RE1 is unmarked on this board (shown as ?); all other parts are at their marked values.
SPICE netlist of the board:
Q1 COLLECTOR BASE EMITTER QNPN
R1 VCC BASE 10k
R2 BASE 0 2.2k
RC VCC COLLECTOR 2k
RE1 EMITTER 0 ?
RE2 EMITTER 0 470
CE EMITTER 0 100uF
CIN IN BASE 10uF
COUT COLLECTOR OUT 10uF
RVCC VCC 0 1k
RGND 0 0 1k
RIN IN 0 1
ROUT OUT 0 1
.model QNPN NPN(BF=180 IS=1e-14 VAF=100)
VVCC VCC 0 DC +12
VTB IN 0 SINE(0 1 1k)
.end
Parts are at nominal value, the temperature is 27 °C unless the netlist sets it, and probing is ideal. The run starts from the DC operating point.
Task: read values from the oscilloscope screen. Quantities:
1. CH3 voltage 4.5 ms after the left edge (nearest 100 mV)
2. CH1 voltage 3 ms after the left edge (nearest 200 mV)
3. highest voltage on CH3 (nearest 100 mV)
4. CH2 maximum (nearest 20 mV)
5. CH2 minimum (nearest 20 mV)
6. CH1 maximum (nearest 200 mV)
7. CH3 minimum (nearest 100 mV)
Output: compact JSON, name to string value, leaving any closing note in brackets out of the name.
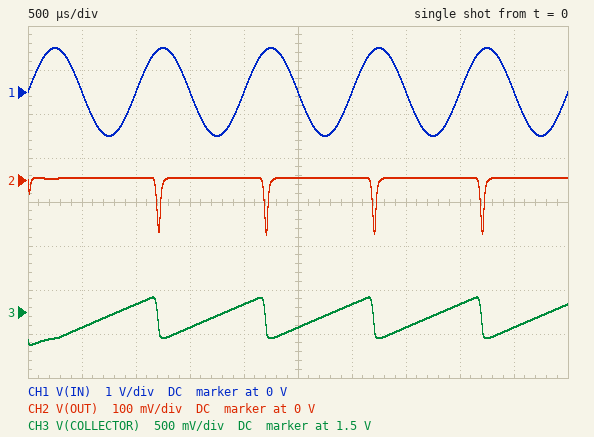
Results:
{"CH3 voltage 4.5 ms after the left edge": "1.3 V", "CH1 voltage 3 ms after the left edge": "0 V", "highest voltage on CH3": "1.7 V", "CH2 maximum": "0 V", "CH2 minimum": "-120 mV", "CH1 maximum": "1.0 V", "CH3 minimum": "1.1 V"}
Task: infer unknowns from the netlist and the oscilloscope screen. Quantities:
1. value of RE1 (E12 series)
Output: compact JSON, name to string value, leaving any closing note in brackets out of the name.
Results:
{"value of RE1": "330 Ω"}
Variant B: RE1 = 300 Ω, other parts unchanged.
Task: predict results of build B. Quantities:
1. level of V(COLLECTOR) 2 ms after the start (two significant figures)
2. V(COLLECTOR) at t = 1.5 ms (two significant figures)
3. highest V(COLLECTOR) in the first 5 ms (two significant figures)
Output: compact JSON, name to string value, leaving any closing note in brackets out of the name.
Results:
{"level of V(COLLECTOR) 2 ms after the start": "1.5 V", "V(COLLECTOR) at t = 1.5 ms": "1.3 V", "highest V(COLLECTOR) in the first 5 ms": "1.6 V"}
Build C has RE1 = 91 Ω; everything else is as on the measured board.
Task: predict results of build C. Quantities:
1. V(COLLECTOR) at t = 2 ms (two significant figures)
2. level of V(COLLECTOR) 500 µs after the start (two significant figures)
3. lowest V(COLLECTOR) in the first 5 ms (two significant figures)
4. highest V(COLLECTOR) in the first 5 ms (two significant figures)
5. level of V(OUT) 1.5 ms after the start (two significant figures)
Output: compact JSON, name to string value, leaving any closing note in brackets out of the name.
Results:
{"V(COLLECTOR) at t = 2 ms": "990 mV", "level of V(COLLECTOR) 500 µs after the start": "720 mV", "lowest V(COLLECTOR) in the first 5 ms": "510 mV", "highest V(COLLECTOR) in the first 5 ms": "1.1 V", "level of V(OUT) 1.5 ms after the start": "5.6 mV"}
